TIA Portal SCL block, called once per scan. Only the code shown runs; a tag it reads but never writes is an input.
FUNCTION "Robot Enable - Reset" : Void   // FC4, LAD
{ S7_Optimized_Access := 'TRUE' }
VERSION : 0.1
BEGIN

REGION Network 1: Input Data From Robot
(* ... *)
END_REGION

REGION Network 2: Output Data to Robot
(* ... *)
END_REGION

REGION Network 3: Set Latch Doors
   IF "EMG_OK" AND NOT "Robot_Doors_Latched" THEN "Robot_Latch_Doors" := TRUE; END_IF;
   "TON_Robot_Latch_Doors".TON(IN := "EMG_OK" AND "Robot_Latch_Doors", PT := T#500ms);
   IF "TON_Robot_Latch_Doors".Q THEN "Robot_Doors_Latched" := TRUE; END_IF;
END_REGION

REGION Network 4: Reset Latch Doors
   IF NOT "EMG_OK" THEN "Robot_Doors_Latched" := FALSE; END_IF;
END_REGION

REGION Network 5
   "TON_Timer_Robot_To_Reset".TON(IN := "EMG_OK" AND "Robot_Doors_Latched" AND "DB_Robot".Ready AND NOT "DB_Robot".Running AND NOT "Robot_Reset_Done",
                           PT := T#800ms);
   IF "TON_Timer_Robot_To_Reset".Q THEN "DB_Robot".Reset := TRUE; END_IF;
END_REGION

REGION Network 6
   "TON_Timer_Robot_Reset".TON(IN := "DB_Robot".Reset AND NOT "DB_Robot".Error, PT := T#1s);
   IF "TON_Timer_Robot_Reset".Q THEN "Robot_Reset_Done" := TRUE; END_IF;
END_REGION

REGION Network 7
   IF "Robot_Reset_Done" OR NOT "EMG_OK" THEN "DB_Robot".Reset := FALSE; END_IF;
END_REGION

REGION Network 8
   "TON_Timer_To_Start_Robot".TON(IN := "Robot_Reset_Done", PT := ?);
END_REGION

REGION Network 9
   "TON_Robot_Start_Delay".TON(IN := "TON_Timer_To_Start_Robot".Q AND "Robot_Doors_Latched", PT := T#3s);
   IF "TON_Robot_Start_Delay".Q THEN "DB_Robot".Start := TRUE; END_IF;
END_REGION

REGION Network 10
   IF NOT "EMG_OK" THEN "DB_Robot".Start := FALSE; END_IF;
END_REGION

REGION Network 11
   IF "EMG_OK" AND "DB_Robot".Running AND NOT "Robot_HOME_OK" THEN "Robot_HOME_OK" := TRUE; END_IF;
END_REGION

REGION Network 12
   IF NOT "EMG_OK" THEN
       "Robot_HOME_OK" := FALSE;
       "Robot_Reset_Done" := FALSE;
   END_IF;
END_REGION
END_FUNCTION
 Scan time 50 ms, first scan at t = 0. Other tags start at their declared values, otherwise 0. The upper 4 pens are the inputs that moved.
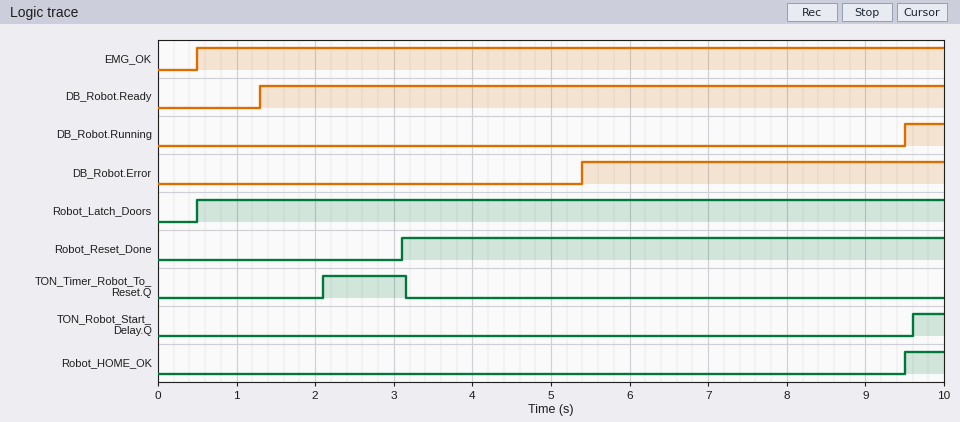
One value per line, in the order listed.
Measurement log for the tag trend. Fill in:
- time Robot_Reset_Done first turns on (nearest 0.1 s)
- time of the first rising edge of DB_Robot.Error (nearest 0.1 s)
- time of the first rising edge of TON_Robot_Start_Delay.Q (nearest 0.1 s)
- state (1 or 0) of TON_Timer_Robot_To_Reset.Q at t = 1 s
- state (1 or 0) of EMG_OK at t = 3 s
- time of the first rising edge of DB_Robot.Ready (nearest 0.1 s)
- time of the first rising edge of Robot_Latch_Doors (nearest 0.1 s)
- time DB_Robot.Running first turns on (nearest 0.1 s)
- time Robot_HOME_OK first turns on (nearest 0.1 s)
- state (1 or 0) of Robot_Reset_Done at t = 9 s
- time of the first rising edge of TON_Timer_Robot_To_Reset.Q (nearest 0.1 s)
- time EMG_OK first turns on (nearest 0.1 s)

3.1 s
5.4 s
9.6 s
0
1
1.3 s
0.5 s
9.5 s
9.5 s
1
2.1 s
0.5 s
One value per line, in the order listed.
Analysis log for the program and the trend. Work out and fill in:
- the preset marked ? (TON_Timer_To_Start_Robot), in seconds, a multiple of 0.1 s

3.5 s
